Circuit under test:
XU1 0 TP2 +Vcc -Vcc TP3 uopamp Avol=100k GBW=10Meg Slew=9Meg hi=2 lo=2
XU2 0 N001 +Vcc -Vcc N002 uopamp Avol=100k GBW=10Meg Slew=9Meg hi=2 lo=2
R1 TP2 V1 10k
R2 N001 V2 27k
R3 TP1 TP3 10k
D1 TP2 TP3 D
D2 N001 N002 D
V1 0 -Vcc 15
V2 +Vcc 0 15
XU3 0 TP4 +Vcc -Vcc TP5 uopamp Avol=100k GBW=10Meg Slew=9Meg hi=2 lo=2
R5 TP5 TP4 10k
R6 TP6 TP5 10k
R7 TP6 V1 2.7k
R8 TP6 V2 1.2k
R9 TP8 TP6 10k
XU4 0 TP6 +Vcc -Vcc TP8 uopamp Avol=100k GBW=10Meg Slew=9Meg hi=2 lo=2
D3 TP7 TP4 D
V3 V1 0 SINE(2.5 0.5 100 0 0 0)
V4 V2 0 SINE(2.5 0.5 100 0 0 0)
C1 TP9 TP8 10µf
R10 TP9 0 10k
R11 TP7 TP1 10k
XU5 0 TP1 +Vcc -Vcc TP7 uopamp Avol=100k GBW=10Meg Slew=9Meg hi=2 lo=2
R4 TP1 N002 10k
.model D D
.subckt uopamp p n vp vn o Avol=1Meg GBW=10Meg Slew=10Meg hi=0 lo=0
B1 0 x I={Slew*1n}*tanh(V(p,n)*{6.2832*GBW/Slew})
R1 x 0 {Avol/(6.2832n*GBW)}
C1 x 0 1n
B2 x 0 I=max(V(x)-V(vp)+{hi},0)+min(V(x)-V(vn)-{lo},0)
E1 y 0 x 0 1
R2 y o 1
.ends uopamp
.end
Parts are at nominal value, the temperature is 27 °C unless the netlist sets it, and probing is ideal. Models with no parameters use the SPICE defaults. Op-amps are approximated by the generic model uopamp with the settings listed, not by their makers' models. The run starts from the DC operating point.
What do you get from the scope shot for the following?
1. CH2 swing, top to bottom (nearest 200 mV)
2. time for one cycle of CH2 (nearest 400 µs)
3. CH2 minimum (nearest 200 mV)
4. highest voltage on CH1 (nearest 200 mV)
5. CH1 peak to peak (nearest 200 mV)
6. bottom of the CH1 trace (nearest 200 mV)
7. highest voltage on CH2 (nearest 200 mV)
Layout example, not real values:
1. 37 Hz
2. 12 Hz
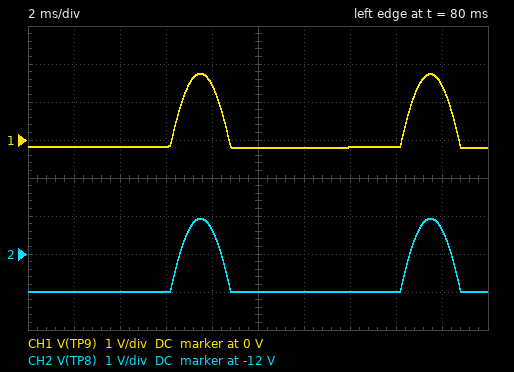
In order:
1. 2.0 V
2. 10.0 ms
3. -13.0 V
4. 1.8 V
5. 2.0 V
6. -200 mV
7. -11.0 V
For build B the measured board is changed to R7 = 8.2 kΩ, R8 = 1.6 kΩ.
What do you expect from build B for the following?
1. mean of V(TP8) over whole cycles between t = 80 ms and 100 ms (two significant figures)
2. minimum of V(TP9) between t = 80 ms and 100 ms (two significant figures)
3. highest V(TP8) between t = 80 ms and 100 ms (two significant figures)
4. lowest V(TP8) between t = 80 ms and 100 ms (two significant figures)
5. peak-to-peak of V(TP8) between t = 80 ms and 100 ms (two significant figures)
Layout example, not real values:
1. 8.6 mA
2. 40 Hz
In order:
1. -5.7 V
2. -3.7 V
3. -1.9 V
4. -9.4 V
5. 7.5 V
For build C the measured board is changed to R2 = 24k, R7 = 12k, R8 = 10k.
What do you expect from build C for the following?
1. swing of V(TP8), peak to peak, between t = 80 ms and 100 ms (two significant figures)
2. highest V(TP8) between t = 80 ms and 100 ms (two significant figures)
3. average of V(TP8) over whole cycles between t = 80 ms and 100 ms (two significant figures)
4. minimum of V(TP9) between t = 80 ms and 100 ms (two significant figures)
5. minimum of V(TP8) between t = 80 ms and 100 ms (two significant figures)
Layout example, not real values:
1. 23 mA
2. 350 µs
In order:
1. 1.8 V
2. 9.3 V
3. 8.4 V
4. -910 mV
5. 7.5 V
